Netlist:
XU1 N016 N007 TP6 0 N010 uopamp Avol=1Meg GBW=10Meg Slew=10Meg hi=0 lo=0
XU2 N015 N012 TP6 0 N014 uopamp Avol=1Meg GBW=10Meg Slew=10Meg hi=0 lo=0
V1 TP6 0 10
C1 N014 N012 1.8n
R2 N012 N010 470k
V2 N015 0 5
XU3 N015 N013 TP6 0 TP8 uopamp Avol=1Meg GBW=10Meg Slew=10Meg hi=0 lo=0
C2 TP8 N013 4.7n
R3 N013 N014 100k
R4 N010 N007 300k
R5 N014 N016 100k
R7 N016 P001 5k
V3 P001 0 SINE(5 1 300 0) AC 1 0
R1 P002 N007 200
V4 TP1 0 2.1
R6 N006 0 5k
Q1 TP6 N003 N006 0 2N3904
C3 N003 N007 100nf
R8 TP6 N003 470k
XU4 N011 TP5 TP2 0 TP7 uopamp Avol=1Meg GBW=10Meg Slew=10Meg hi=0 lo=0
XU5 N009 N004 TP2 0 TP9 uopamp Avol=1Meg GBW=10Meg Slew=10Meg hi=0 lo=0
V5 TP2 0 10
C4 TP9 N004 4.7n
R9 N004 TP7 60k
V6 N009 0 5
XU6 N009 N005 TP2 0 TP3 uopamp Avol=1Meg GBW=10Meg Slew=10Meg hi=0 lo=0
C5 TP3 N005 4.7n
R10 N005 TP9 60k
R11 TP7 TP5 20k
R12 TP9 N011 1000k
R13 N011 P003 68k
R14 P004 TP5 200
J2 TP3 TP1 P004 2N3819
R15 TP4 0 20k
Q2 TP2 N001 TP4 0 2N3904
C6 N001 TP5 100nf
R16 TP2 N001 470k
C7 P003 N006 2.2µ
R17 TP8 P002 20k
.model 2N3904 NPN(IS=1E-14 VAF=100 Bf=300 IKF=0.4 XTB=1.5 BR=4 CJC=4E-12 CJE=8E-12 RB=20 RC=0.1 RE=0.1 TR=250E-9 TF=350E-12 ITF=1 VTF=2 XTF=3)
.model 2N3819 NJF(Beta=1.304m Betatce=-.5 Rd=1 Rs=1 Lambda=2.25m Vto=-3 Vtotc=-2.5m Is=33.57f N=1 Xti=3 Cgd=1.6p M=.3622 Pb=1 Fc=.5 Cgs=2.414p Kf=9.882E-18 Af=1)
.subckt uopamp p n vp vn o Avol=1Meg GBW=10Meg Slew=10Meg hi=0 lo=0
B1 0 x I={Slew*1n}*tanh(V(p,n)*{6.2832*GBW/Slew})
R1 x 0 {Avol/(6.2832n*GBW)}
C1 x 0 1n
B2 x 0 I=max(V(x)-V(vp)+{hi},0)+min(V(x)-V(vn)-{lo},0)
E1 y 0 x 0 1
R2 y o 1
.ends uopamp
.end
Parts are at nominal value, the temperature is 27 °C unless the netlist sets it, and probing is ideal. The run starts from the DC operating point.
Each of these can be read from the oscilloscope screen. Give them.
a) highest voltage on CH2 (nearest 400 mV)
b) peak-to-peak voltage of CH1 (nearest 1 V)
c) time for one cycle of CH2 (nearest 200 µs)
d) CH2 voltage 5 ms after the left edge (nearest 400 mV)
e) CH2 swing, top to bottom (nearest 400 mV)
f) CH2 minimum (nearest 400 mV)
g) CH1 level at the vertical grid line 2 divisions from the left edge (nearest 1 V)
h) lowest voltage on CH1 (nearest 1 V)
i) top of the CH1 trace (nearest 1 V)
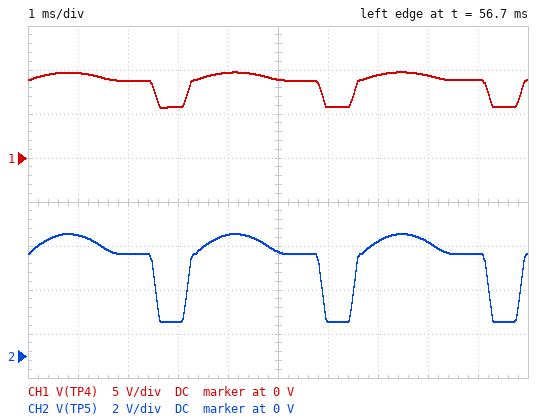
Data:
5.6 V
4 V
3.4 ms
4.8 V
4.0 V
1.6 V
9 V
6 V
10 V
